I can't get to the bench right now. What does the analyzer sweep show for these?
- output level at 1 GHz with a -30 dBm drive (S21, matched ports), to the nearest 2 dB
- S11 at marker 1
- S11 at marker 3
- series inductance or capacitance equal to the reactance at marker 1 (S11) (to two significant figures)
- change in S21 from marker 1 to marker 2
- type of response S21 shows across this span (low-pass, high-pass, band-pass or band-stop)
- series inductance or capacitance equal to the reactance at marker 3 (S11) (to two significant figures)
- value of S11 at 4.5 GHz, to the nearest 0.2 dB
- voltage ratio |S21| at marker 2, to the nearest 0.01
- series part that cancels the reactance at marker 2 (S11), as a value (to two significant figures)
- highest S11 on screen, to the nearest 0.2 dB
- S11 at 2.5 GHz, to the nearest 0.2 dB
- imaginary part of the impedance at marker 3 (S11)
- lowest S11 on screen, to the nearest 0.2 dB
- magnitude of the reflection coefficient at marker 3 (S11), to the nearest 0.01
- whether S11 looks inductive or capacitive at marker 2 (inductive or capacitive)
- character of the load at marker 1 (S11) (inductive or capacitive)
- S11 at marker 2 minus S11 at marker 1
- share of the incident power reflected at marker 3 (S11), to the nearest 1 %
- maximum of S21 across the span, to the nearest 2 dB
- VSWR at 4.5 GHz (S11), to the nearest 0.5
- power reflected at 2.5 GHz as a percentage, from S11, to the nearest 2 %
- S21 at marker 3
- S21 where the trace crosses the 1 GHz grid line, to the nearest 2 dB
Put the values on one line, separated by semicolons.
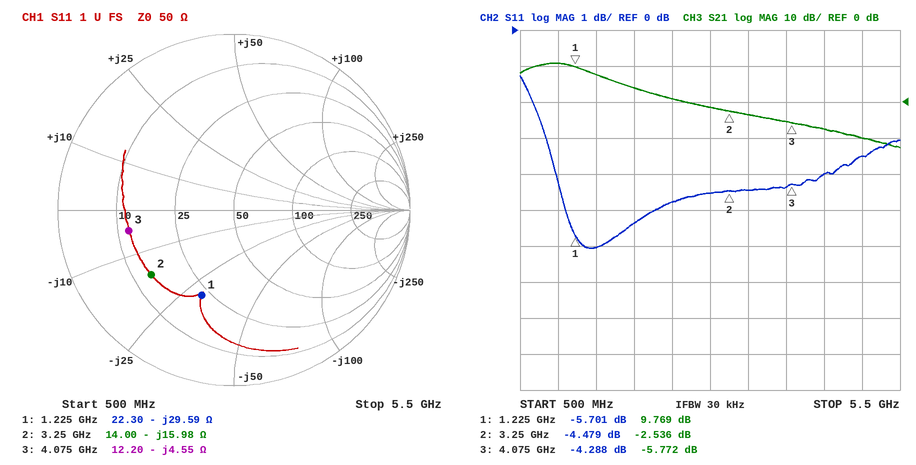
-20 dBm; -5.701 dB; -4.288 dB; 4.4 pF; -12.305 dB; low-pass; 8.6 pF; -4.0 dB; 0.75; 780 pH; -1.2 dB; -4.8 dB; -4.55 Ω; -6.0 dB; 0.61; capacitive; capacitive; 1.222 dB; 37 %; 10 dB; 4.5; 34 %; -5.772 dB; 10 dB
